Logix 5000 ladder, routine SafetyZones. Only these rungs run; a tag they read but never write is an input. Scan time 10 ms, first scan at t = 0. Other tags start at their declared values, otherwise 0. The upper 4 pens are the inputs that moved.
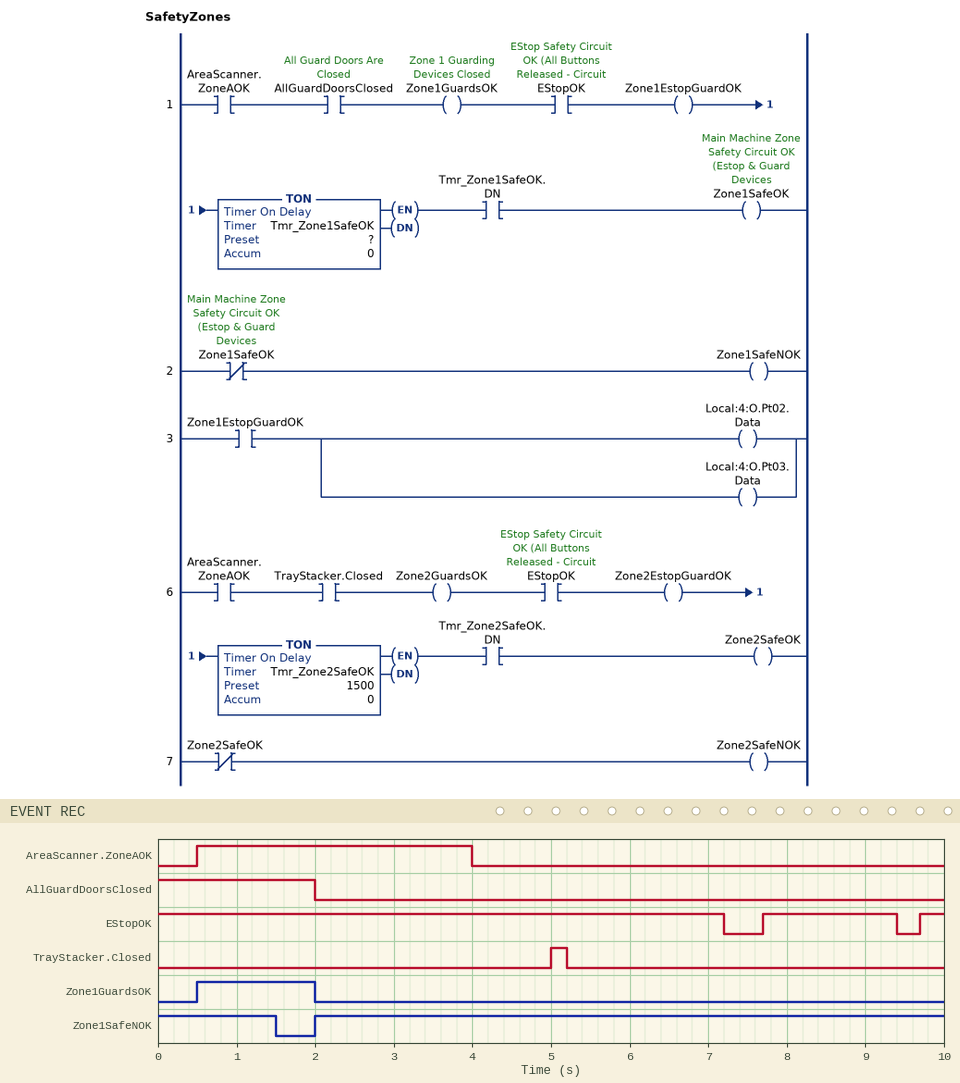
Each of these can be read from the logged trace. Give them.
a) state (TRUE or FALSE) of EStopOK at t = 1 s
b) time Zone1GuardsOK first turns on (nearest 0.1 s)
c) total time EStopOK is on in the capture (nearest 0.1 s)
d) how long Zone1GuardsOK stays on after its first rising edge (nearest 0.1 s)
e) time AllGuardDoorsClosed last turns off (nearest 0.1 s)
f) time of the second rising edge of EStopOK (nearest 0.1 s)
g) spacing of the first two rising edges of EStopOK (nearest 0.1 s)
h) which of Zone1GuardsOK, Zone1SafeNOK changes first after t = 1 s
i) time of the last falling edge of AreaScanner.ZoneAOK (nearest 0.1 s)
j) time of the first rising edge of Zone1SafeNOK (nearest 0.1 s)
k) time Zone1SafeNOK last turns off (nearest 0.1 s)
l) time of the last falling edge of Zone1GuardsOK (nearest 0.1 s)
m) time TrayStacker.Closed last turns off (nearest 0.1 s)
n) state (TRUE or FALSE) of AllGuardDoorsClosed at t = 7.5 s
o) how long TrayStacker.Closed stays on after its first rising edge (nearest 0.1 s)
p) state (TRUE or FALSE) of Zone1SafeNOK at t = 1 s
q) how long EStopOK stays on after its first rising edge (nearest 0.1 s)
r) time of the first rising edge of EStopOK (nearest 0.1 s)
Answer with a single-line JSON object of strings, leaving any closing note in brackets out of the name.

{"state (TRUE or FALSE) of EStopOK at t = 1 s": "TRUE", "time Zone1GuardsOK first turns on": "0.5 s", "total time EStopOK is on in the capture": "9.2 s", "how long Zone1GuardsOK stays on after its first rising edge": "1.5 s", "time AllGuardDoorsClosed last turns off": "2.0 s", "time of the second rising edge of EStopOK": "9.7 s", "spacing of the first two rising edges of EStopOK": "2.0 s", "which of Zone1GuardsOK, Zone1SafeNOK changes first after t = 1 s": "Zone1SafeNOK", "time of the last falling edge of AreaScanner.ZoneAOK": "4.0 s", "time of the first rising edge of Zone1SafeNOK": "2.0 s", "time Zone1SafeNOK last turns off": "1.5 s", "time of the last falling edge of Zone1GuardsOK": "2.0 s", "time TrayStacker.Closed last turns off": "5.2 s", "state (TRUE or FALSE) of AllGuardDoorsClosed at t = 7.5 s": "FALSE", "how long TrayStacker.Closed stays on after its first rising edge": "0.2 s", "state (TRUE or FALSE) of Zone1SafeNOK at t = 1 s": "TRUE", "how long EStopOK stays on after its first rising edge": "1.7 s", "time of the first rising edge of EStopOK": "7.7 s"}
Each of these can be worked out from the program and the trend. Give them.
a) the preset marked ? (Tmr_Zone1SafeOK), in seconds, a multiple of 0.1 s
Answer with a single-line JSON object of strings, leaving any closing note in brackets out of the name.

{"the preset marked ? (Tmr_Zone1SafeOK), in seconds, a multiple of 0.1 s": "1.0 s"}
